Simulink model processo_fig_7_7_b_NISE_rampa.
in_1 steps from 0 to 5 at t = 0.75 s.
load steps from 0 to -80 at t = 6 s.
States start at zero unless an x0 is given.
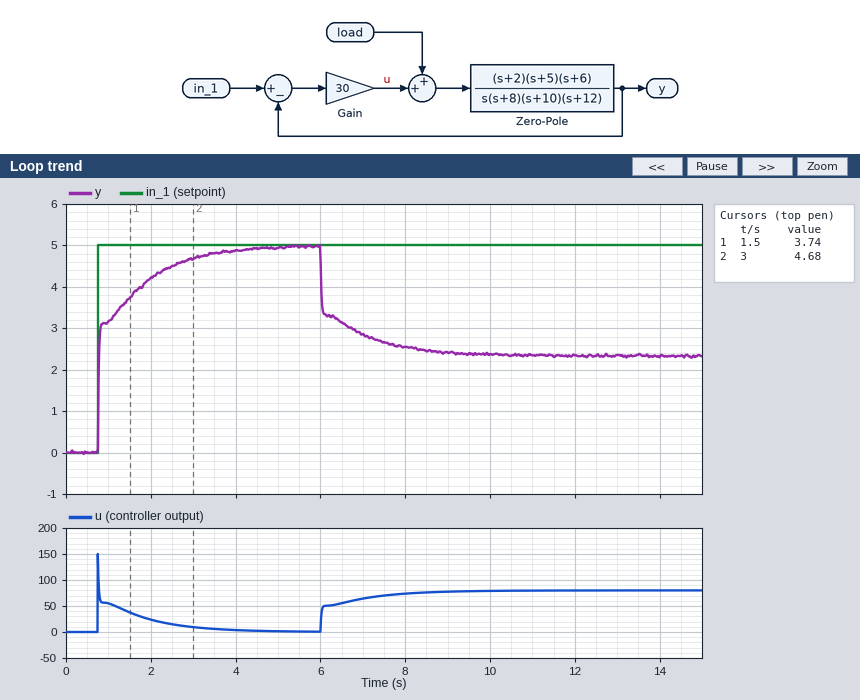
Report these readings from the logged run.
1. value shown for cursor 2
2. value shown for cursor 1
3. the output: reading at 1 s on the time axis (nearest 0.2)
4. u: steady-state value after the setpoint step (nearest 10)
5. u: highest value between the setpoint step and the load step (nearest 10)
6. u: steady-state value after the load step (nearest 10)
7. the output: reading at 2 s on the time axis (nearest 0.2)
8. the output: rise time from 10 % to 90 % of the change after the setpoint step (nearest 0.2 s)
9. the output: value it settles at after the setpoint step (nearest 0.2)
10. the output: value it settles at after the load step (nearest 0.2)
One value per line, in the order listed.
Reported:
4.68
3.74
3.2
0
150
80
4.2
1.8 s
5.0
2.4
